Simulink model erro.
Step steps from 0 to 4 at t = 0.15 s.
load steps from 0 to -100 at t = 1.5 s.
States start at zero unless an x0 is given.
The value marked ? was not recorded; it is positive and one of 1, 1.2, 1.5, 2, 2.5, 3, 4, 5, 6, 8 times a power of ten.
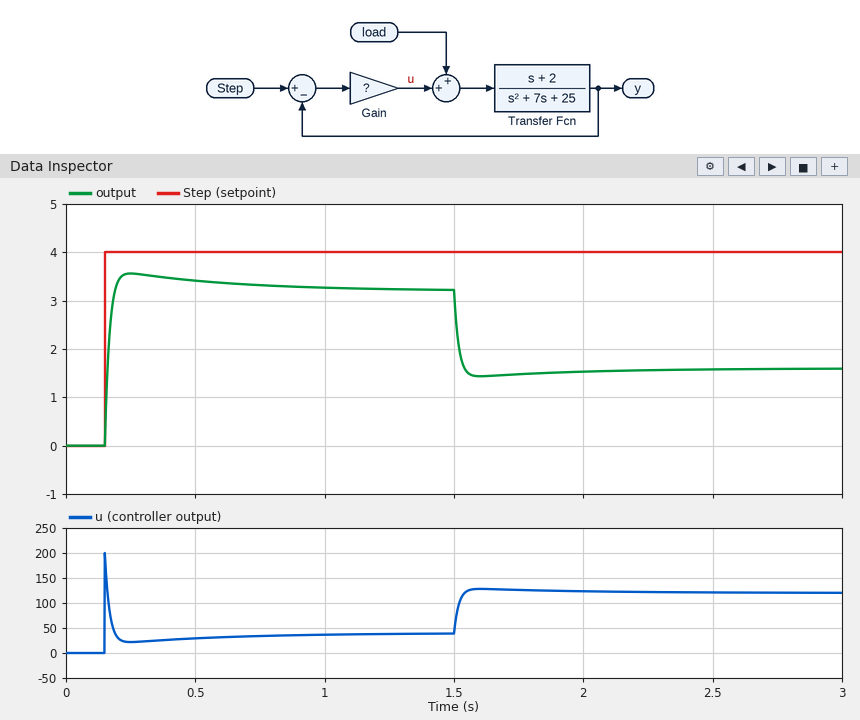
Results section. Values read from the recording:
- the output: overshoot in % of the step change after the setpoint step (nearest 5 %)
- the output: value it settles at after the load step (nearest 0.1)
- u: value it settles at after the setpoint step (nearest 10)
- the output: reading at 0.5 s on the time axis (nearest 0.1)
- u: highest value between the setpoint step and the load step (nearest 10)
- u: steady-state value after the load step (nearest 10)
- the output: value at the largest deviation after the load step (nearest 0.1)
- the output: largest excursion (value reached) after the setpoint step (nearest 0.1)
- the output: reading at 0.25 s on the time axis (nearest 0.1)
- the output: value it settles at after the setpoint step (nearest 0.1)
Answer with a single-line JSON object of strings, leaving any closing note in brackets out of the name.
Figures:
{"the output: overshoot in % of the step change after the setpoint step": "10 %", "the output: value it settles at after the load step": "1.6", "u: value it settles at after the setpoint step": "40", "the output: reading at 0.5 s on the time axis": "3.4", "u: highest value between the setpoint step and the load step": "200", "u: steady-state value after the load step": "120", "the output: value at the largest deviation after the load step": "1.4", "the output: largest excursion (value reached) after the setpoint step": "3.6", "the output: reading at 0.25 s on the time axis": "3.6", "the output: value it settles at after the setpoint step": "3.2"}
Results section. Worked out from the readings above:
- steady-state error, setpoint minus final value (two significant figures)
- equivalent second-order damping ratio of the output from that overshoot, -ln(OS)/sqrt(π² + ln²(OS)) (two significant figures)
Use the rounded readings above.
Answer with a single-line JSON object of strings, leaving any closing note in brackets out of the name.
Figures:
{"steady-state error, setpoint minus final value": "0.80", "equivalent second-order damping ratio of the output from that overshoot, -ln(OS)/sqrt(π² + ln²(OS))": "0.59"}
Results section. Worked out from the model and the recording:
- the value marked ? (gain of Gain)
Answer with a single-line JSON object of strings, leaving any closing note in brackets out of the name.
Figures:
{"the value marked ?": "50"}
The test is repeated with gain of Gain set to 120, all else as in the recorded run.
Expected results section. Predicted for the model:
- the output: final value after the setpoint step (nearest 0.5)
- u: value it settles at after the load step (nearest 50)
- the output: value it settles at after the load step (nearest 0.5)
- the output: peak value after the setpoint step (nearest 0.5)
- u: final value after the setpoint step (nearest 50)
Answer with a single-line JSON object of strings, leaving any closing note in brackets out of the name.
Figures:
{"the output: final value after the setpoint step": "3.5", "u: value it settles at after the load step": "150", "the output: value it settles at after the load step": "3.0", "the output: peak value after the setpoint step": "4.0", "u: final value after the setpoint step": "50"}
